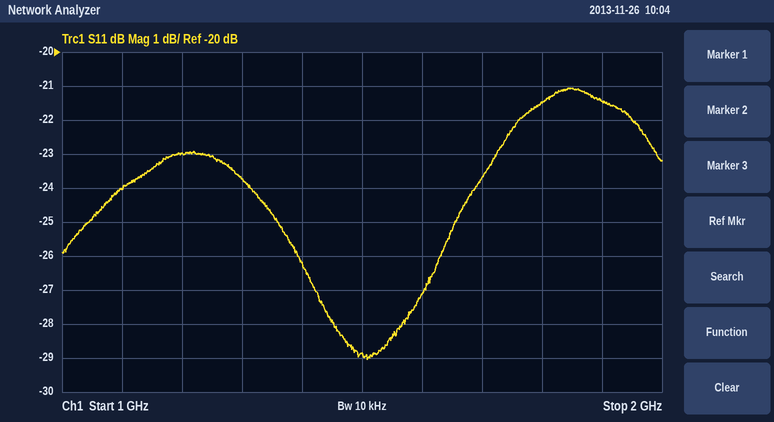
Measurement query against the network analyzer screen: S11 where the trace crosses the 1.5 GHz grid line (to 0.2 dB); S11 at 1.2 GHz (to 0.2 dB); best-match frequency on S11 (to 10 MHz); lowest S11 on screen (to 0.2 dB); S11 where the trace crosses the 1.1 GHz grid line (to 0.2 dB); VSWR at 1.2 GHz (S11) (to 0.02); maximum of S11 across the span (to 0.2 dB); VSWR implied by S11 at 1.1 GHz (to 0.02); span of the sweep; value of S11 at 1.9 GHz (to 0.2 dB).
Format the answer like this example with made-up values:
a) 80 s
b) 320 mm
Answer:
a) -28.8 dB
b) -23.0 dB
c) 1.51 GHz
d) -29.0 dB
e) -24.0 dB
f) 1.16
g) -21.0 dB
h) 1.14
i) 1 GHz
j) -21.4 dB
